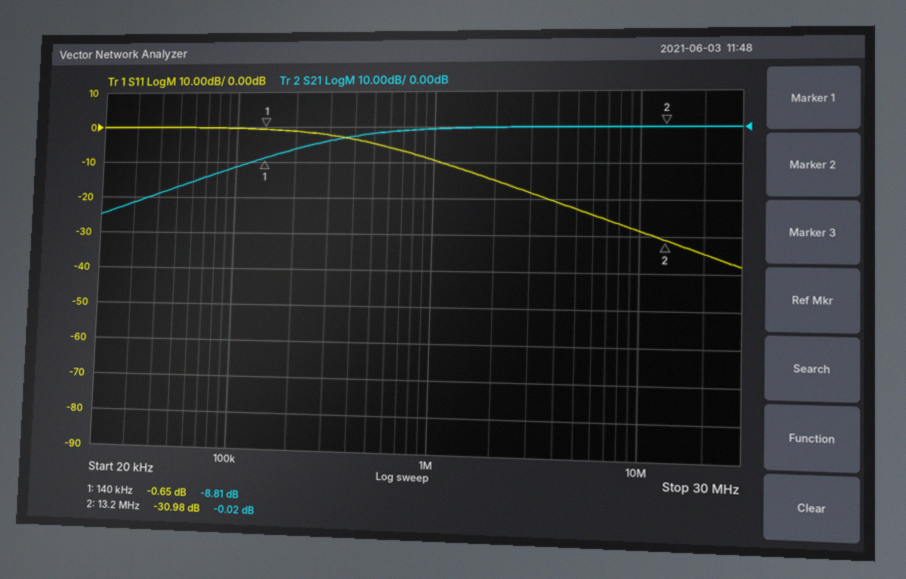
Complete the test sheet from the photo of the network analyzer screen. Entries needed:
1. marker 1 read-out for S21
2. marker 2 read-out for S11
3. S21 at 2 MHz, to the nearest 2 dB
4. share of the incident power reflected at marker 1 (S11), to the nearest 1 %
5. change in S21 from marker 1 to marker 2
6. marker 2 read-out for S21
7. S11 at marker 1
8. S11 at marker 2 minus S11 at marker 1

-8.81 dB
-30.98 dB
0 dB
86 %
8.79 dB
-0.02 dB
-0.65 dB
-30.33 dB
